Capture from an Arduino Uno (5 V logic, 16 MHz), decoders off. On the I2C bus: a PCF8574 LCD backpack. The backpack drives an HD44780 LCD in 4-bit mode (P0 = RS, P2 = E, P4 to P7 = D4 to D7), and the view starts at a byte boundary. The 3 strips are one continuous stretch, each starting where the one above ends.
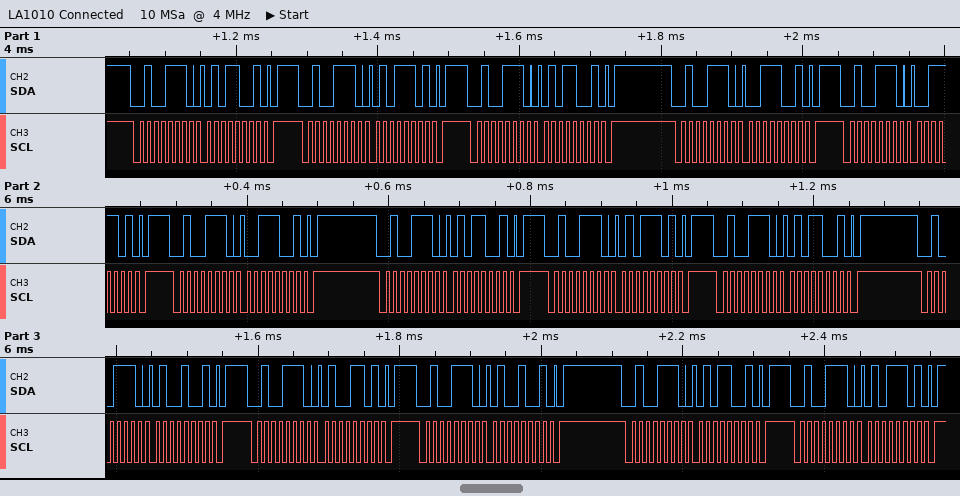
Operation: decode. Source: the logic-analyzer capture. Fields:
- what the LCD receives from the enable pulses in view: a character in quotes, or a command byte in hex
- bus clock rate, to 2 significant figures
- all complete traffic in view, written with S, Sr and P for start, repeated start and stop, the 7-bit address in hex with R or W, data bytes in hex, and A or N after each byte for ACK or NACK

'S' 'T'
100 kHz
S 27W A 59 A P S 27W A 5D A P S 27W A 59 A P S 27W A 39 A P S 27W A 3D A P S 27W A 39 A P S 27W A 59 A P S 27W A 5D A P S 27W A 59 A P S 27W A 49 A P S 27W A 4D A P S 27W A 49 A P S 27W A 59 A P S 27W A 5D A P
